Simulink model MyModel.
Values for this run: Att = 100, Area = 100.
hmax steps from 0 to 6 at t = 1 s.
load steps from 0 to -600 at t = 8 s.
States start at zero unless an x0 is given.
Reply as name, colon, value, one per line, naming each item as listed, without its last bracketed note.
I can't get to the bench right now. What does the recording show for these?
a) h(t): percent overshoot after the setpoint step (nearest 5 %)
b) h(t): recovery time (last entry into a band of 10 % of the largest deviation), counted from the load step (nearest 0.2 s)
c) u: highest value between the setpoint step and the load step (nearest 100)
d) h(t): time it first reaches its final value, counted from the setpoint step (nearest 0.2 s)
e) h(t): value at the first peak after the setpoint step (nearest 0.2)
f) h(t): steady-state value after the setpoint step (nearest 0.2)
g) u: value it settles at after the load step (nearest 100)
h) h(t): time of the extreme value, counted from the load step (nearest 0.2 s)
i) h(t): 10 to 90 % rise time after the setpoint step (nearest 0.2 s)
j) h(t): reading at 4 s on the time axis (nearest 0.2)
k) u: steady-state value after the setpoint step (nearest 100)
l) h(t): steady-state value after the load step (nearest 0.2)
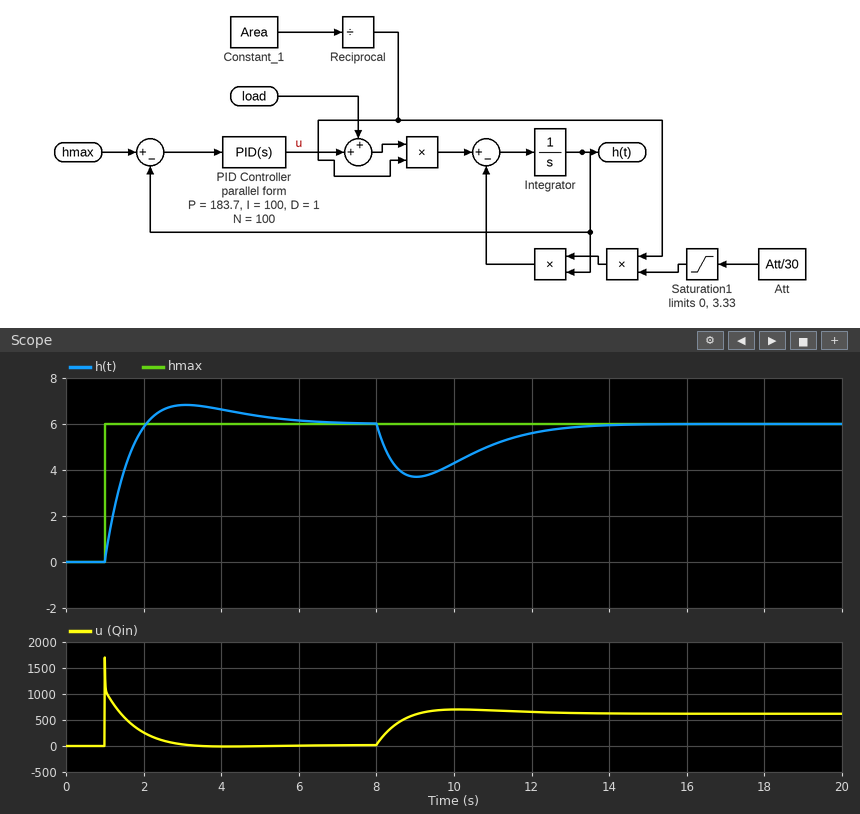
h(t): percent overshoot after the setpoint step: 15 %
h(t): recovery time (last entry into a band of 10 % of the largest deviation), counted from the load step: 4.6 s
u: highest value between the setpoint step and the load step: 1700
h(t): time it first reaches its final value, counted from the setpoint step: 1.0 s
h(t): value at the first peak after the setpoint step: 6.8
h(t): steady-state value after the setpoint step: 6.0
u: value it settles at after the load step: 600
h(t): time of the extreme value, counted from the load step: 1.0 s
h(t): 10 to 90 % rise time after the setpoint step: 0.8 s
h(t): reading at 4 s on the time axis: 6.6
u: steady-state value after the setpoint step: 0
h(t): steady-state value after the load step: 6.0
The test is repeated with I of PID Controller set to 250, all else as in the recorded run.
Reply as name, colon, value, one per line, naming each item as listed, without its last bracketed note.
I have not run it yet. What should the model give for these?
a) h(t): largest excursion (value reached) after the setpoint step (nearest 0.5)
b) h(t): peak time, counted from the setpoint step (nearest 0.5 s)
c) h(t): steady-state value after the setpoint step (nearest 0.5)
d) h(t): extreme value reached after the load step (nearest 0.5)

h(t): largest excursion (value reached) after the setpoint step: 7.5
h(t): peak time, counted from the setpoint step: 1.5 s
h(t): steady-state value after the setpoint step: 6.0
h(t): extreme value reached after the load step: 4.0
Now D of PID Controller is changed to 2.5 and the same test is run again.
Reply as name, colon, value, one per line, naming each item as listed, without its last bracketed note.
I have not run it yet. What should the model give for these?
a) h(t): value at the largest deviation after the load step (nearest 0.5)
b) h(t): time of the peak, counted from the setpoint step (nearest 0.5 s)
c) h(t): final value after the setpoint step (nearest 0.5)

h(t): value at the largest deviation after the load step: 3.5
h(t): time of the peak, counted from the setpoint step: 2.0 s
h(t): final value after the setpoint step: 6.0
